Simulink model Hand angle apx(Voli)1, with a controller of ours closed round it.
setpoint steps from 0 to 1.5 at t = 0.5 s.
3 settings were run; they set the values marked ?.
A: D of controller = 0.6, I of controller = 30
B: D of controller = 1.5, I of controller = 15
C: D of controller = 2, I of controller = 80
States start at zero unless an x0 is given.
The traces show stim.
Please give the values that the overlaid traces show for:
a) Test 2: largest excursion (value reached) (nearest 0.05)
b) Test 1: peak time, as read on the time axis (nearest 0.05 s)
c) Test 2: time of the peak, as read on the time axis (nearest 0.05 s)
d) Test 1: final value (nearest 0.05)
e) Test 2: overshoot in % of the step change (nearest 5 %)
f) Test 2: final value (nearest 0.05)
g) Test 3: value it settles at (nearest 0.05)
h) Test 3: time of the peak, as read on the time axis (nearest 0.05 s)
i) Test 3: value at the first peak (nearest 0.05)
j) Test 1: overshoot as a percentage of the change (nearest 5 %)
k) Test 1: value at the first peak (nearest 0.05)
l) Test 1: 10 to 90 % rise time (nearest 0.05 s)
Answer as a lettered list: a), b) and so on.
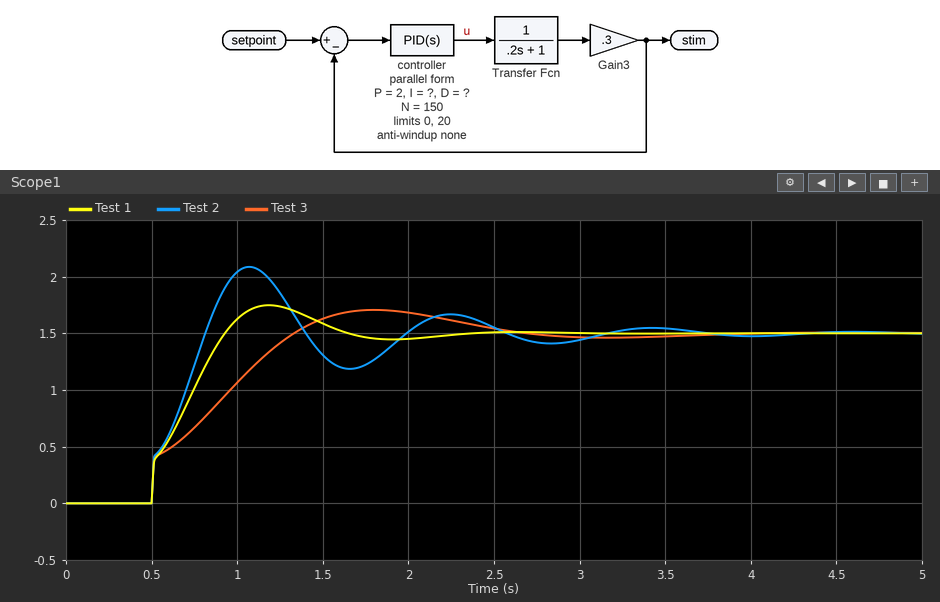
a) 2.10
b) 1.20 s
c) 1.05 s
d) 1.50
e) 40 %
f) 1.50
g) 1.50
h) 1.80 s
i) 1.70
j) 15 %
k) 1.75
l) 0.35 s
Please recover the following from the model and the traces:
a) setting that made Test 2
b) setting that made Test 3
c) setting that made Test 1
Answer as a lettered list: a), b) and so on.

a) C
b) B
c) A
